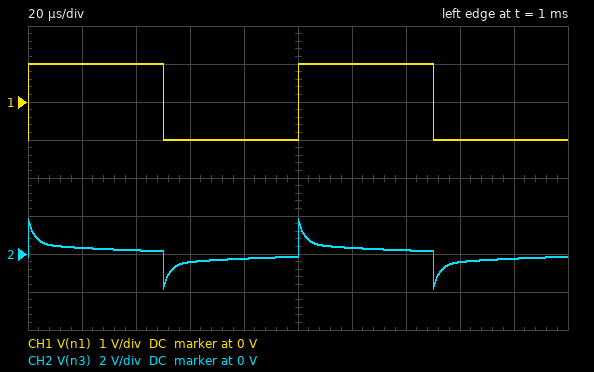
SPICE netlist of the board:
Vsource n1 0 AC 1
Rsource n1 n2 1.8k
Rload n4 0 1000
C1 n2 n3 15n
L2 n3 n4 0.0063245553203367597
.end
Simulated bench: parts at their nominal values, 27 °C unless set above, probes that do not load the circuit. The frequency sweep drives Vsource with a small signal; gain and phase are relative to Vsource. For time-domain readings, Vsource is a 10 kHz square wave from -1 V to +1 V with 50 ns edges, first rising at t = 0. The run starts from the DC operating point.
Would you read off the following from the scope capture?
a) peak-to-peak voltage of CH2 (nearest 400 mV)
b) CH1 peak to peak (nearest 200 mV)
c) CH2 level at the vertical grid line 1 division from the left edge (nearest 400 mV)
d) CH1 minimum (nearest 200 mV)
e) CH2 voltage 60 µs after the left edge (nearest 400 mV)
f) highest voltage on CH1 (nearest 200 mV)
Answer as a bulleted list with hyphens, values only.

- 3.6 V
- 2.0 V
- 400 mV
- -1.0 V
- -400 mV
- 1.0 V
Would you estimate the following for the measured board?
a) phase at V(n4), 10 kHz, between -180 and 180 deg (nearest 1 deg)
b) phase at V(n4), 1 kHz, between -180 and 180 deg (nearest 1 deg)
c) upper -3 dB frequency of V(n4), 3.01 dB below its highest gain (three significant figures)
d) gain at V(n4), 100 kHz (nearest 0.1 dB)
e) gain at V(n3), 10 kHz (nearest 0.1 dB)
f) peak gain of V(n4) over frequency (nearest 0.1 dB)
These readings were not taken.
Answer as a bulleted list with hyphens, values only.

- 13 deg
- 75 deg
- 74.1 kHz
- -13.6 dB
- -8.5 dB
- -8.9 dB
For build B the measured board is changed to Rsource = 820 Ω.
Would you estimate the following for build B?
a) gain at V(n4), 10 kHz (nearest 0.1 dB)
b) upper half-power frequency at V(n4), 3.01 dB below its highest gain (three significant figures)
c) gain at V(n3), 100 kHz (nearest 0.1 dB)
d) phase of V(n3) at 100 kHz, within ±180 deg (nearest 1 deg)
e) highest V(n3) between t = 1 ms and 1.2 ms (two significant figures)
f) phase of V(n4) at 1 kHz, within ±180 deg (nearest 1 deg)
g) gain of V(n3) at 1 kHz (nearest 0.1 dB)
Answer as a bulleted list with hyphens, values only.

- -5.7 dB
- 51.0 kHz
- -0.4 dB
- 11 deg
- 1.9 V
- 80 deg
- -20.6 dB
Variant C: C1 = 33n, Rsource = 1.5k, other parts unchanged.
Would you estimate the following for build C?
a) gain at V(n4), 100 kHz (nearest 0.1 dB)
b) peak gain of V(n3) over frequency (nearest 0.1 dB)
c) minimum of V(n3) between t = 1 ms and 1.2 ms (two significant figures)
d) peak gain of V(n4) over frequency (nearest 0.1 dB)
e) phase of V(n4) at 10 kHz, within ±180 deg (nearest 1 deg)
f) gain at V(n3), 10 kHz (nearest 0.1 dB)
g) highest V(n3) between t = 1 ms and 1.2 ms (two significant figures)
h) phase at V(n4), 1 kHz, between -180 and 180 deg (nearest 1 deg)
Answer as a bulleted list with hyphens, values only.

- -13.4 dB
- 0 dB
- -1.7 V
- -8.0 dB
- 2 deg
- -7.3 dB
- 1.7 V
- 62 deg
